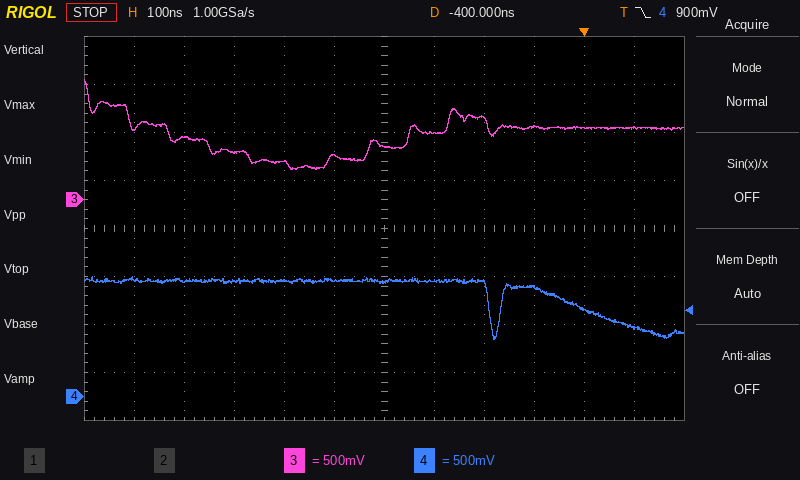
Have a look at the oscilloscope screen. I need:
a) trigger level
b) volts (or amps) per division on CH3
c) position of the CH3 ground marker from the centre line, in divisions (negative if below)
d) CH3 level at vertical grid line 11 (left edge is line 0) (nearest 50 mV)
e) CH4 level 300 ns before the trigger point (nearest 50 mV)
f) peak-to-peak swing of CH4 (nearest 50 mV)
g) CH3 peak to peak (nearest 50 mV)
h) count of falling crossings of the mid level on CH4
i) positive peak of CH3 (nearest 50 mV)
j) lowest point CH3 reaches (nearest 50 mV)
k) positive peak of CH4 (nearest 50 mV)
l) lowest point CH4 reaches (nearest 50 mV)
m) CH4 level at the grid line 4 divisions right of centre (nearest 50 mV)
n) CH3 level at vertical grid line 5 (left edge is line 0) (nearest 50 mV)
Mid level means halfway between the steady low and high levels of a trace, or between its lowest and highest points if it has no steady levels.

900 mV
500 mV
+0.6 div
750 mV
1.20 V
650 mV
950 mV
2
1.25 V
300 mV
1.25 V
600 mV
900 mV
450 mV
